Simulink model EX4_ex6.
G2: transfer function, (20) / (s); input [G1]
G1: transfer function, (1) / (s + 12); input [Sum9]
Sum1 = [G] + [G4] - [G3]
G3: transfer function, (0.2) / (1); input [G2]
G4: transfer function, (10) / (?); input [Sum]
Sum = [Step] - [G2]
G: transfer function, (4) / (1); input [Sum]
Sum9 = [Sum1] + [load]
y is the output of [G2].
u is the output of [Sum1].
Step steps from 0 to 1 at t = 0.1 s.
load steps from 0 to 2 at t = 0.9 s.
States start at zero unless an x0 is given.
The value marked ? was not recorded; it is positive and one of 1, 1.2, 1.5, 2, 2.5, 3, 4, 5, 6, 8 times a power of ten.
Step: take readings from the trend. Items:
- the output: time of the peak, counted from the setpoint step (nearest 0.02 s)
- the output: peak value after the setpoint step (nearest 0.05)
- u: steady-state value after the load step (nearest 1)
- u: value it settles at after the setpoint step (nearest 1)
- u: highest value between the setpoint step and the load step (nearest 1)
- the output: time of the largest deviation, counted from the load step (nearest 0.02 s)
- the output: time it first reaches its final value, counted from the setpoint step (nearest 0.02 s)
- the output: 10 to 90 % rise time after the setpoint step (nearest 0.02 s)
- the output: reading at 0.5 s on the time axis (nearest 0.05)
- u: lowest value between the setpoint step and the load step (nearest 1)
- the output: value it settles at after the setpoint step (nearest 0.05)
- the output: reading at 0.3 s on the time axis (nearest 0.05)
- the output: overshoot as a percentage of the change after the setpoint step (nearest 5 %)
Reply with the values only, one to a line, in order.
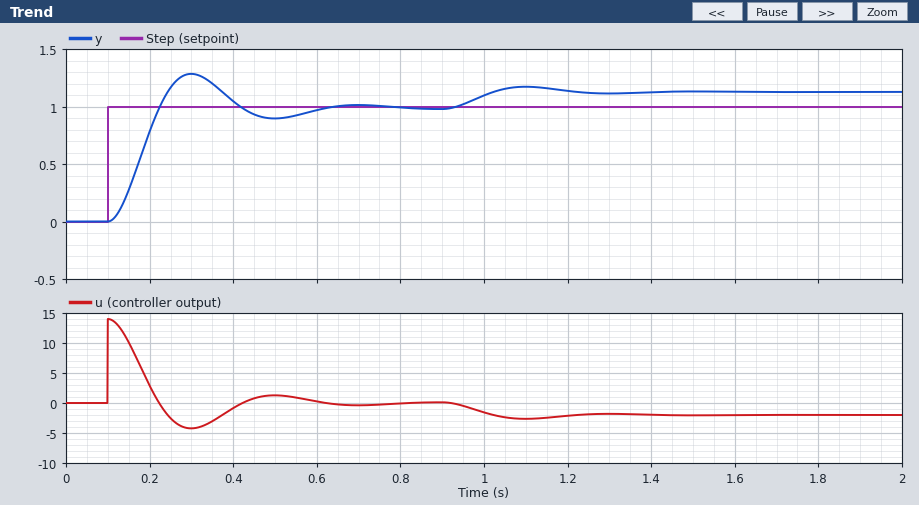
0.20 s
1.30
-2
0
14
0.20 s
0.12 s
0.08 s
0.90
-4
1.00
1.30
30 %
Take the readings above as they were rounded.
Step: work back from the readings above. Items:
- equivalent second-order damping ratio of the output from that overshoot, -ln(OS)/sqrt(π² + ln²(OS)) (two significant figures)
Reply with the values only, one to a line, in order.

0.36
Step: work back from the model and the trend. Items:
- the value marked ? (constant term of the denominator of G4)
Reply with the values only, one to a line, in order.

1
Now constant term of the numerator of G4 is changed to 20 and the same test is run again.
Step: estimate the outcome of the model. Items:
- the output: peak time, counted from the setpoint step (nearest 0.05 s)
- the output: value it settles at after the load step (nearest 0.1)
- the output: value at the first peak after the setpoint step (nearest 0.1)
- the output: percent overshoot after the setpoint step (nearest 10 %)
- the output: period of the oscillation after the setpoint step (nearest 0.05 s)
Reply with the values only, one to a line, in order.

0.15 s
1.1
1.4
40 %
0.30 s
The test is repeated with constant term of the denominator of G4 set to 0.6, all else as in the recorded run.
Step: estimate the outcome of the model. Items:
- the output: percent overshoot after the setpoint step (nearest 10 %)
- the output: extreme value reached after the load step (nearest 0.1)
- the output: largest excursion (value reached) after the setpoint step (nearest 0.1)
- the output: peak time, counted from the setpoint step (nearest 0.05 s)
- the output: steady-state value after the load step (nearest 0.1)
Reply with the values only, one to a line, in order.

40 %
1.1
1.4
0.15 s
1.1
